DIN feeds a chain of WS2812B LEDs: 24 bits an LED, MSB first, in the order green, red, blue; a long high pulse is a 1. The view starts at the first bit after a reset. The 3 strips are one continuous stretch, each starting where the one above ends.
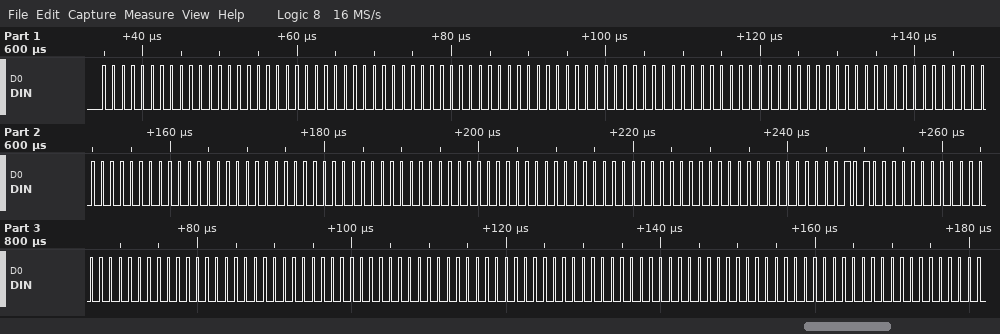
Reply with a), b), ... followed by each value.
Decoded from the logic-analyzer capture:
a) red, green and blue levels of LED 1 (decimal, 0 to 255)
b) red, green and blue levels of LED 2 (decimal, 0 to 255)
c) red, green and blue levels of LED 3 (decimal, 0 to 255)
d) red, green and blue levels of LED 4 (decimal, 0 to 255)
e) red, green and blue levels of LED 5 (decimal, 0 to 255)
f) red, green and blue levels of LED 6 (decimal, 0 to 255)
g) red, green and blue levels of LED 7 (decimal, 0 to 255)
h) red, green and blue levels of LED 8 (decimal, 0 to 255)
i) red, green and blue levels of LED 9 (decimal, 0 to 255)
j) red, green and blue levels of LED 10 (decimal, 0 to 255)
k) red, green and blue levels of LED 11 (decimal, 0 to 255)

a) 0, 0, 0
b) 0, 0, 0
c) 0, 0, 0
d) 0, 0, 0
e) 0, 0, 0
f) 0, 0, 0
g) 0, 0, 0
h) 0, 40, 0
i) 0, 0, 0
j) 0, 0, 0
k) 0, 0, 0
